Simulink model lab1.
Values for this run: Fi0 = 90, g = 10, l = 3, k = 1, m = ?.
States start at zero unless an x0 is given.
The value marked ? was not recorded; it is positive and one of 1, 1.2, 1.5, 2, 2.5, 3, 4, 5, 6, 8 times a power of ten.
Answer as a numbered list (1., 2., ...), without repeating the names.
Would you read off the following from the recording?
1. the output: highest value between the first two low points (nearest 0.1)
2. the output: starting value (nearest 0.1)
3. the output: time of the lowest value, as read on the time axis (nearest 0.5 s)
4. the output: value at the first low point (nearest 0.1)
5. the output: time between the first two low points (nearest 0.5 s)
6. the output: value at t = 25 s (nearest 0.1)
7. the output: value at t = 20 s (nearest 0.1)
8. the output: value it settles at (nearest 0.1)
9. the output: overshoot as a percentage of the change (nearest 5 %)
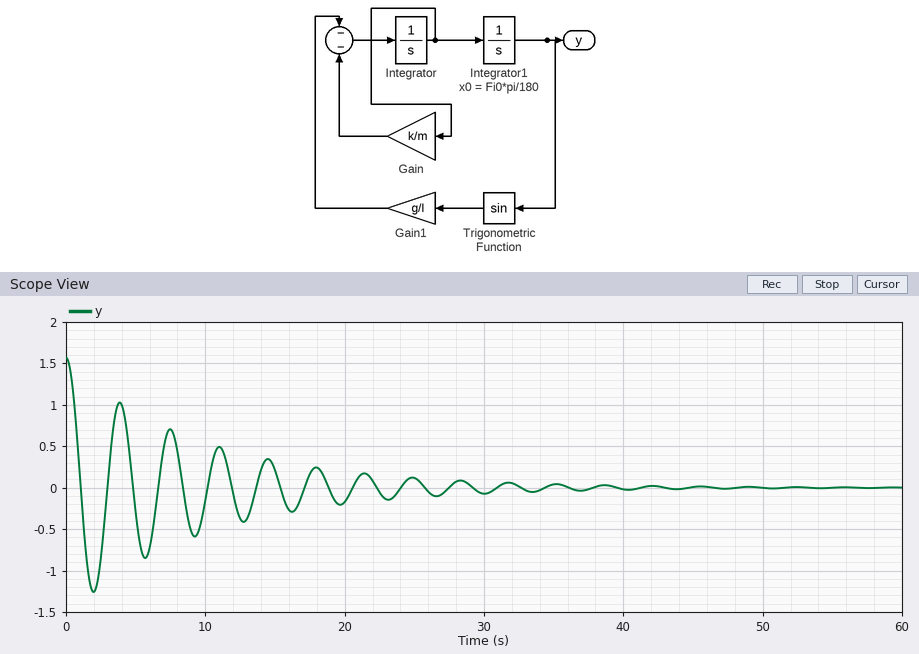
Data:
1. 1.0
2. 1.6
3. 2.0 s
4. -1.3
5. 3.5 s
6. 0.1
7. -0.2
8. 0.0
9. 80 %
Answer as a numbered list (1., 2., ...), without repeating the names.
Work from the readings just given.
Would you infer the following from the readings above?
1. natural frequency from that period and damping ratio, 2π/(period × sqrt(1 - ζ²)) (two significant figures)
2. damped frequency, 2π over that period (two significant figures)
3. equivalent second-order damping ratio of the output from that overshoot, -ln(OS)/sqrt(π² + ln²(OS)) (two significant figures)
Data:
1. 1.8 rad/s
2. 1.8 rad/s
3. 0.071
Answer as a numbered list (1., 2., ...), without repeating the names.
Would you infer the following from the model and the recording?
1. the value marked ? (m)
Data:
1. 5
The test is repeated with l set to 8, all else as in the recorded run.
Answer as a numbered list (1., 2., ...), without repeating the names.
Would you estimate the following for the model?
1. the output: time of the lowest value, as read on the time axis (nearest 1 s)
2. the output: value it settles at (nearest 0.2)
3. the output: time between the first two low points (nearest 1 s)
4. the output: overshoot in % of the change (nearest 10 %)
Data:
1. 3 s
2. 0.0
3. 6 s
4. 70 %
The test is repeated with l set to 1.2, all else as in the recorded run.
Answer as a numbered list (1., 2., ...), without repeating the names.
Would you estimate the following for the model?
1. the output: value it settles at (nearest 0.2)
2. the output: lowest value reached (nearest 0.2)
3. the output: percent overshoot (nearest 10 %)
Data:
1. 0.0
2. -1.4
3. 90 %
